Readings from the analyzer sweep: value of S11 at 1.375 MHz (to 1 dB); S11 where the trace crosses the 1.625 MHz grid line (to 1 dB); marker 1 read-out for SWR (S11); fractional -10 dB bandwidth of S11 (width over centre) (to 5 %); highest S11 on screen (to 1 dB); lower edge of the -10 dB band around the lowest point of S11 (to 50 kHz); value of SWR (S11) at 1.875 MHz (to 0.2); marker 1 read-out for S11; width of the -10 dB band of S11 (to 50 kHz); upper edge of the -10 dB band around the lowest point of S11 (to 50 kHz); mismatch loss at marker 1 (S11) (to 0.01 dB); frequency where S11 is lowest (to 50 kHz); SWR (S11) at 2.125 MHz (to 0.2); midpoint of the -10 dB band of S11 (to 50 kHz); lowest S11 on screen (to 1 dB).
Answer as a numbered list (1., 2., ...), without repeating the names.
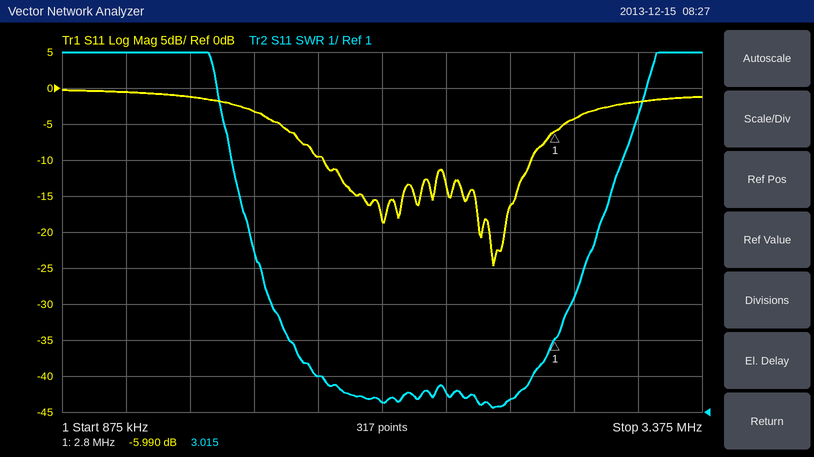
1. -1 dB
2. -3 dB
3. 3.015
4. 35 %
5. 0 dB
6. 1.90 MHz
7. 2.0
8. -5.990 dB
9. 800 kHz
10. 2.70 MHz
11. 1.26 dB
12. 2.55 MHz
13. 1.2
14. 2.30 MHz
15. -25 dB
